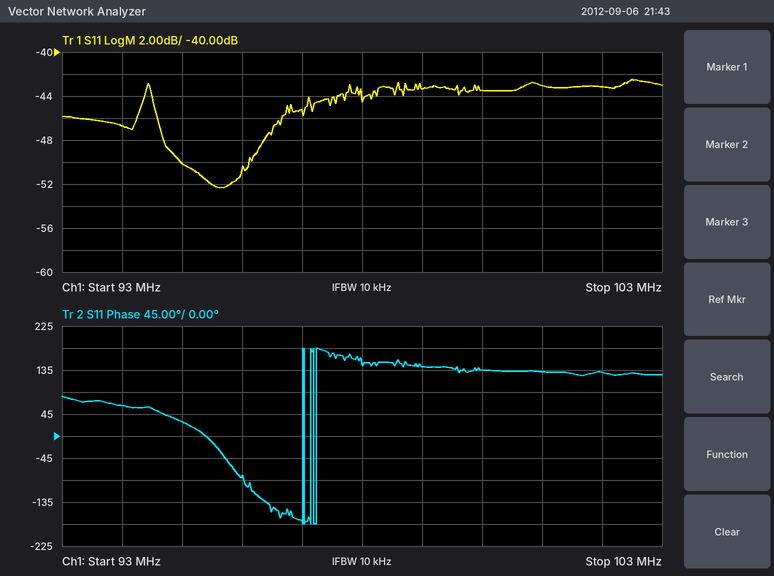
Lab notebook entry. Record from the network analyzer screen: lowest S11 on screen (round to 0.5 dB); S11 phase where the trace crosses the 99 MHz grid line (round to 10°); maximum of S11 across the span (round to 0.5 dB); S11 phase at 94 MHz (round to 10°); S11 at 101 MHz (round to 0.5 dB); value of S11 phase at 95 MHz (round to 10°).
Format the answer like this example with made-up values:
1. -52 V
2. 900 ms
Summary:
1. -52.5 dB
2. 140°
3. -42.5 dB
4. 60°
5. -43.0 dB
6. 30°
